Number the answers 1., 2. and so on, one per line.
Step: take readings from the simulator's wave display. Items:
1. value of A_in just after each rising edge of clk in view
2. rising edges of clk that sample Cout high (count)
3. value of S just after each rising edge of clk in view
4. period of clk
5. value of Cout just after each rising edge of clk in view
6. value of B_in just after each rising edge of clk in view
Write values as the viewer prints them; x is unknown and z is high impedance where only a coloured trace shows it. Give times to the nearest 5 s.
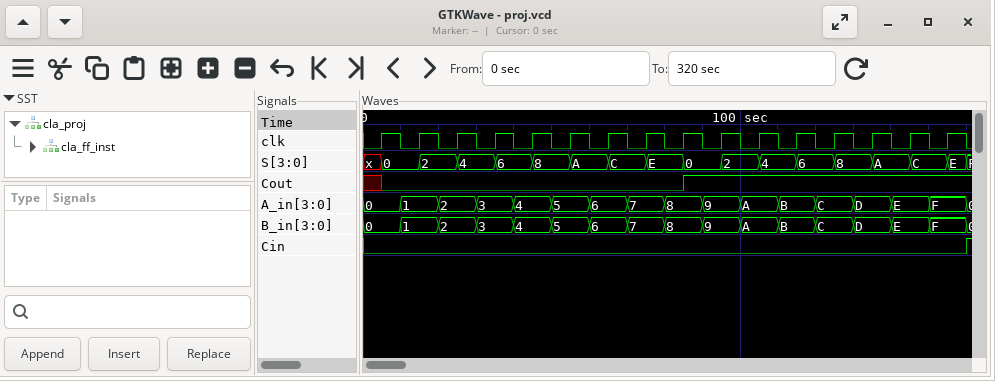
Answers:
1. 0, 1, 2, 3, 4, 5, 6, 7, 8, 9, A, B, C, D, E, F
2. 7
3. 0, 2, 4, 6, 8, A, C, E, 0, 2, 4, 6, 8, A, C, E
4. 10 s
5. 0 0 0 0 0 0 0 0 1 1 1 1 1 1 1 1
6. 0, 1, 2, 3, 4, 5, 6, 7, 8, 9, A, B, C, D, E, F
